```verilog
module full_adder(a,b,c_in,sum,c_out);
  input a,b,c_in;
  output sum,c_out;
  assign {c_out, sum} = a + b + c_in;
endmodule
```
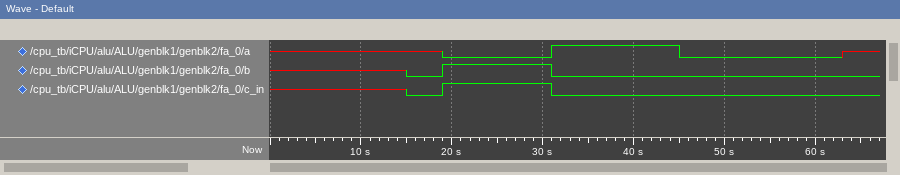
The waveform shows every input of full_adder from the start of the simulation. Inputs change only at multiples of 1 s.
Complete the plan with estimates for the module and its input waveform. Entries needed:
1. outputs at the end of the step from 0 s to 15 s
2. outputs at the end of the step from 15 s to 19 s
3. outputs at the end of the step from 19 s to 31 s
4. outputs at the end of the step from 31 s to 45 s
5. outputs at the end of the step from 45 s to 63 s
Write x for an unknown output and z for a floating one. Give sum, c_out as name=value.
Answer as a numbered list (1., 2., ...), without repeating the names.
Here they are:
1. sum=x, c_out=x
2. sum=x, c_out=x
3. sum=0, c_out=1
4. sum=1, c_out=0
5. sum=0, c_out=0
